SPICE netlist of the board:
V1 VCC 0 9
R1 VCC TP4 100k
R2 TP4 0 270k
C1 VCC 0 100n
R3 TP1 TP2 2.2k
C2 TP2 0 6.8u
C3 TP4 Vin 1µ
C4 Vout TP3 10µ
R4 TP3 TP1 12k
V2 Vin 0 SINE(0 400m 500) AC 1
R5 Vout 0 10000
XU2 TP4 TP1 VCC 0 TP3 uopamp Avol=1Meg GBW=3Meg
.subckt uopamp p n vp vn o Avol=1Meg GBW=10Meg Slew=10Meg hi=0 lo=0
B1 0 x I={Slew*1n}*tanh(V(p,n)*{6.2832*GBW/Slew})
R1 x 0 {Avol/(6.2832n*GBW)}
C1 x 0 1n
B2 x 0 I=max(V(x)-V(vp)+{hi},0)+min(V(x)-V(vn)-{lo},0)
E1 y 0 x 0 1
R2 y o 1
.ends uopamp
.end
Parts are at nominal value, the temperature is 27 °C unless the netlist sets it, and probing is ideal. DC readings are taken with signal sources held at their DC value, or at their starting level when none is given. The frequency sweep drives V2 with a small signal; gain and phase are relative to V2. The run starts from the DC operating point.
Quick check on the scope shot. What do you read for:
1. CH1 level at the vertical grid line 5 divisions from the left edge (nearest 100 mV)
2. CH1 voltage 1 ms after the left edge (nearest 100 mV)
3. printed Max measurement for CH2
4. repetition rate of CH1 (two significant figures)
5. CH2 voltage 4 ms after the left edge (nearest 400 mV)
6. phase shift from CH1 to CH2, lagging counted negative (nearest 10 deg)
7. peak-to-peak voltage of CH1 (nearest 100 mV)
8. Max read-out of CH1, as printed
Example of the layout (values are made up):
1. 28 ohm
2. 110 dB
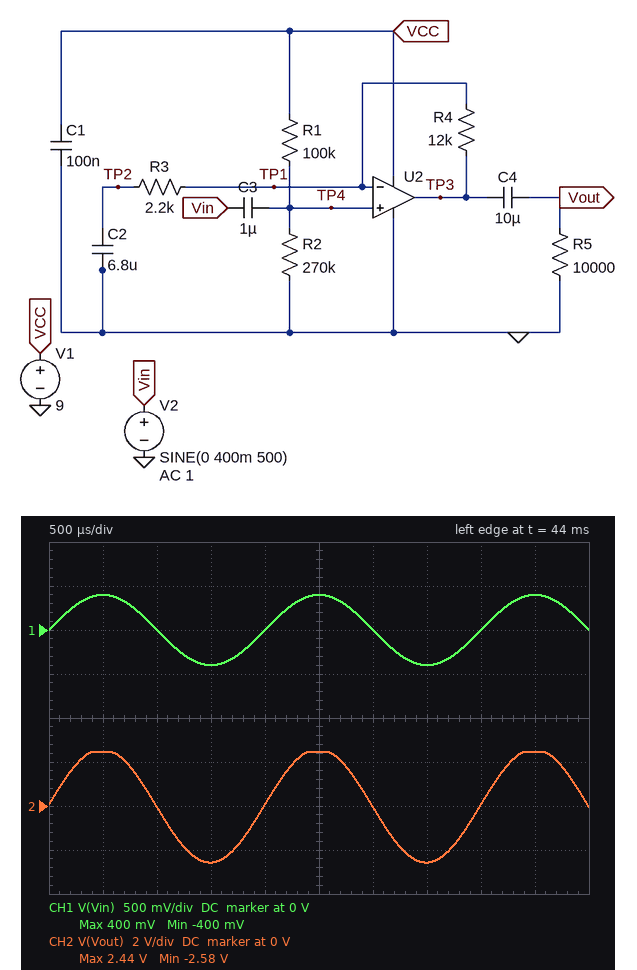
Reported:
1. 400 mV
2. 0 V
3. 2.44 V
4. 500 Hz
5. 0 V
6. 0 deg
7. 800 mV
8. 400 mV
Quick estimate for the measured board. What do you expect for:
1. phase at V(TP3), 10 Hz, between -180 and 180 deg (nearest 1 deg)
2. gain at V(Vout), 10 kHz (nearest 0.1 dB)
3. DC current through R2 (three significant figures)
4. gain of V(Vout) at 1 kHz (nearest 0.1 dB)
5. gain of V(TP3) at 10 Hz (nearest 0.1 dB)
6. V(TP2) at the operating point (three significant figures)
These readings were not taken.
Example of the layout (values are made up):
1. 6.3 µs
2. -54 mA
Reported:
1. 50 deg
2. 16.2 dB
3. 24.3 µA
4. 16.2 dB
5. 12.8 dB
6. 6.57 V
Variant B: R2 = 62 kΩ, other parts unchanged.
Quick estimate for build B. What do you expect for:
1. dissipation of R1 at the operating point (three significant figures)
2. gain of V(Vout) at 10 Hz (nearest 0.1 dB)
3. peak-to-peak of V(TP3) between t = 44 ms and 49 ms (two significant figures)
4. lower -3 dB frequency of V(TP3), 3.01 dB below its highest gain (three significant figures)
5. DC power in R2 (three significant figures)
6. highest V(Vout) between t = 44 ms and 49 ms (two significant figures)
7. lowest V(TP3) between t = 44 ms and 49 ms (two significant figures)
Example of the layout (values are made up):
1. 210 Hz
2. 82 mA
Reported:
1. 309 µW
2. 12.2 dB
3. 5.2 V
4. 11.8 Hz
5. 191 µW
6. 2.6 V
7. 860 mV
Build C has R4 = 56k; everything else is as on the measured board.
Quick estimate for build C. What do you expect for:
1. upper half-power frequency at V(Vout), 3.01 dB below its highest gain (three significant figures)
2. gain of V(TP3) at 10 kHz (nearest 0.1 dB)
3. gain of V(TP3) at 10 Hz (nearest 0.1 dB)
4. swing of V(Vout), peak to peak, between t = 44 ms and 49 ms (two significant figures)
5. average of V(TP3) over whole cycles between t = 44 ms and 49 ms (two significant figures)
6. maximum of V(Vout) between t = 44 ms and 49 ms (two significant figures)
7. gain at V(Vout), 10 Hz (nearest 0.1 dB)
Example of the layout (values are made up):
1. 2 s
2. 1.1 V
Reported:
1. 113 kHz
2. 28.4 dB
3. 25.0 dB
4. 9.0 V
5. 5.9 V
6. 2.8 V
7. 24.9 dB
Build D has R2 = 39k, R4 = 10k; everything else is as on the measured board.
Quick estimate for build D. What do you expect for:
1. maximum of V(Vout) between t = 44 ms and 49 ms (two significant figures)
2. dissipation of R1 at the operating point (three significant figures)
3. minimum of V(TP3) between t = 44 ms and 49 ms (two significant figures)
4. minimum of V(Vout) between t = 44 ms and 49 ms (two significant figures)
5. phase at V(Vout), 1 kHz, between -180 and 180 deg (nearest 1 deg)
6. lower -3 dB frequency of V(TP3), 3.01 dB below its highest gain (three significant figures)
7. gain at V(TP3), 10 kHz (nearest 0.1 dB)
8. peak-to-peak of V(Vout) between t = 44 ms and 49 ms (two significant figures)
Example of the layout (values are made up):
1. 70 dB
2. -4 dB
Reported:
1. 2.2 V
2. 419 µW
3. 310 mV
4. -2.2 V
5. 1 deg
6. 12.7 Hz
7. 14.9 dB
8. 4.4 V
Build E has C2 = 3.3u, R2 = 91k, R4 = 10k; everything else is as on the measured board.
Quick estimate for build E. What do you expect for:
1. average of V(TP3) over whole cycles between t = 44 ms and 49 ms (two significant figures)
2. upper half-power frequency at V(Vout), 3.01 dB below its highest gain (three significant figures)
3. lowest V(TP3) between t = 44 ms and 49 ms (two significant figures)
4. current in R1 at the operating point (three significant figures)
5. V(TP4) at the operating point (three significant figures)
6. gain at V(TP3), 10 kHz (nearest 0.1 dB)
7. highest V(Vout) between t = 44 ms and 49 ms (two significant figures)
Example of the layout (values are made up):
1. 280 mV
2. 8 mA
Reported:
1. 4.3 V
2. 541 kHz
3. 2.1 V
4. 47.1 µA
5. 4.29 V
6. 14.9 dB
7. 2.2 V
